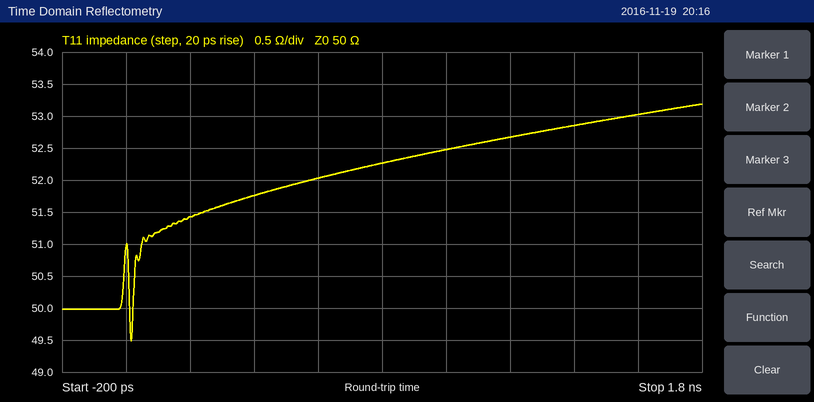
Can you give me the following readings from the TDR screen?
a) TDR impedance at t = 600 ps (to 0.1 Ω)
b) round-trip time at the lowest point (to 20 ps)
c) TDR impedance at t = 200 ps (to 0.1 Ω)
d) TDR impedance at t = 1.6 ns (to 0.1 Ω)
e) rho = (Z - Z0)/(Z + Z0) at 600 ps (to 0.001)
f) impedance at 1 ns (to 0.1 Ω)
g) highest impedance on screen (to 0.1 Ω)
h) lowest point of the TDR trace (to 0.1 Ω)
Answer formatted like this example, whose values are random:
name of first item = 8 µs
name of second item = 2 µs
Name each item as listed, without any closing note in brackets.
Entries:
TDR impedance at t = 600 ps = 52.0 Ω
round-trip time at the lowest point = 20 ps
TDR impedance at t = 200 ps = 51.4 Ω
TDR impedance at t = 1.6 ns = 53.0 Ω
rho = (Z - Z0)/(Z + Z0) at 600 ps = +0.020
impedance at 1 ns = 52.5 Ω
highest impedance on screen = 53.2 Ω
lowest point of the TDR trace = 49.5 Ω
